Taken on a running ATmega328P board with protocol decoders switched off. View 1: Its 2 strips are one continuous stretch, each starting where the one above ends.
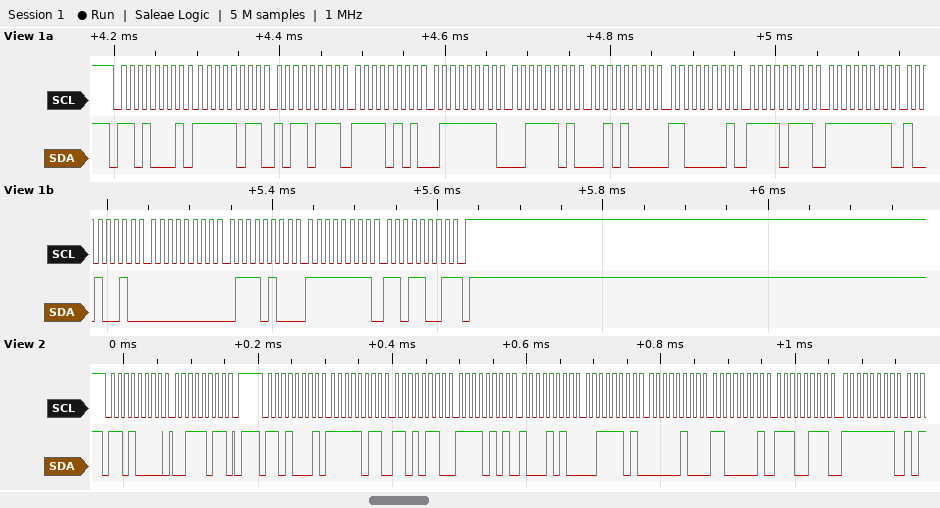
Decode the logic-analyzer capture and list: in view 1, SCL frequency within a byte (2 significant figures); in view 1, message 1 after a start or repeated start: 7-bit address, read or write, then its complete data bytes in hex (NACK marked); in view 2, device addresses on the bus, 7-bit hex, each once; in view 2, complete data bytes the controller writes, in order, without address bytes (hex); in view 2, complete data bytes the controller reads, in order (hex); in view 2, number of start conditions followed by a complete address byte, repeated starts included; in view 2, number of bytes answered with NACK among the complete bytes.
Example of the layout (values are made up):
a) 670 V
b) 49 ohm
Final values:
a) 100 kHz
b) 0x68 read: FB B7 F5 7F 3D 28 C1 F7 FF 92 00 74 FF D9 NACK
c) 0x68
d) 3B
e) FB D6 F5 8A 3D 04 C1 E7 FF
f) 2
g) 0
